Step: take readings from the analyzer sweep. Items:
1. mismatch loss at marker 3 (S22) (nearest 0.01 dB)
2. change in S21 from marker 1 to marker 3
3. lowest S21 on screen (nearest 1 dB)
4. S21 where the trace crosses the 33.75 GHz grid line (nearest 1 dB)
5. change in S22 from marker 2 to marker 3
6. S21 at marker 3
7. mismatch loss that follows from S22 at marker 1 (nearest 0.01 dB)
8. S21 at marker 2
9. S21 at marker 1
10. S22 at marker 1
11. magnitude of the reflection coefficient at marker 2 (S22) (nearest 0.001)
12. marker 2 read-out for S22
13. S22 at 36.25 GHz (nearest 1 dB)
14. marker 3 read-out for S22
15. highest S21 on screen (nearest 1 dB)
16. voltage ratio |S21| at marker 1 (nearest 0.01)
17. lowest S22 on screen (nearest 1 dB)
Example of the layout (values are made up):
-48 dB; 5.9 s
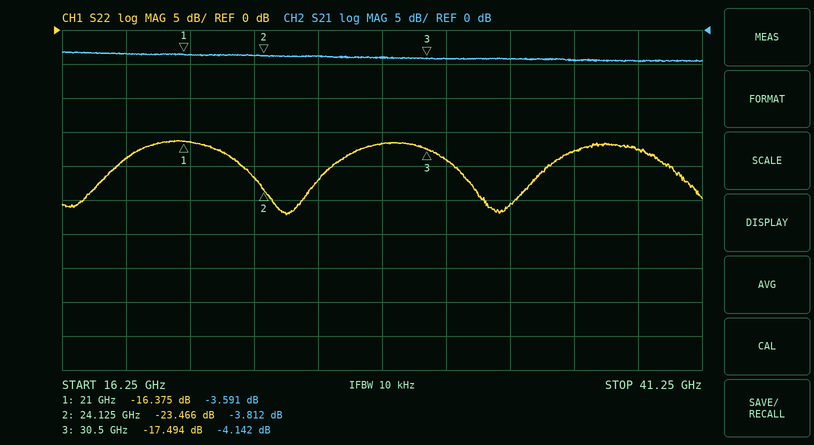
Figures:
0.08 dB; -0.551 dB; -5 dB; -4 dB; 5.972 dB; -4.142 dB; 0.10 dB; -3.812 dB; -3.591 dB; -16.375 dB; 0.067; -23.466 dB; -18 dB; -17.494 dB; -3 dB; 0.66; -27 dB
